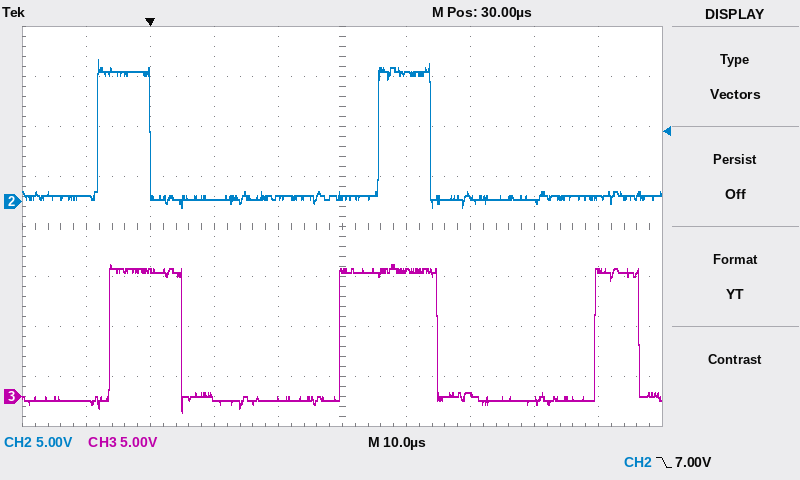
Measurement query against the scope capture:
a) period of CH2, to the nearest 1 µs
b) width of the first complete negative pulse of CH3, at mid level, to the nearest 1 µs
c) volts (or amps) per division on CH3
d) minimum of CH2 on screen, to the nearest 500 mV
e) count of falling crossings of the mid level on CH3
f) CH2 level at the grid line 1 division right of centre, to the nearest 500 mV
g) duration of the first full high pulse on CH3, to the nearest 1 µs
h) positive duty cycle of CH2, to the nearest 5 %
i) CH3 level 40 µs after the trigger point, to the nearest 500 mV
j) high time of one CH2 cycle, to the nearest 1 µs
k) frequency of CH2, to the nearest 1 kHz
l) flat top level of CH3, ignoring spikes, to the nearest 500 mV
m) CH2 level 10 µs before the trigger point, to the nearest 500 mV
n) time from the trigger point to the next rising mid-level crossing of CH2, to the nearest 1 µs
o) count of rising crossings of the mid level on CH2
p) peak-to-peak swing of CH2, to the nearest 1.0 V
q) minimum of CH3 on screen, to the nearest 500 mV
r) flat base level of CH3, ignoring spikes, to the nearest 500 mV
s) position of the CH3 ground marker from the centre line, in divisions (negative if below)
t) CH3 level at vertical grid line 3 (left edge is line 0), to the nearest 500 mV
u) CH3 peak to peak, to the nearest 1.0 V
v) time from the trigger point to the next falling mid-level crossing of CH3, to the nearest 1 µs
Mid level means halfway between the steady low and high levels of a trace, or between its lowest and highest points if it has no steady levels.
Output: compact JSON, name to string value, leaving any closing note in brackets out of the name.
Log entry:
{"period of CH2, to the nearest 1 µs": "44 µs", "width of the first complete negative pulse of CH3, at mid level, to the nearest 1 µs": "25 µs", "volts (or amps) per division on CH3": "5 V", "minimum of CH2 on screen, to the nearest 500 mV": "-500 mV", "count of falling crossings of the mid level on CH3": "3", "CH2 level at the grid line 1 division right of centre, to the nearest 500 mV": "13.0 V", "duration of the first full high pulse on CH3, to the nearest 1 µs": "11 µs", "positive duty cycle of CH2, to the nearest 5 %": "20 %", "CH3 level 40 µs after the trigger point, to the nearest 500 mV": "12.5 V", "high time of one CH2 cycle, to the nearest 1 µs": "8 µs", "frequency of CH2, to the nearest 1 kHz": "23 kHz", "flat top level of CH3, ignoring spikes, to the nearest 500 mV": "12.5 V", "CH2 level 10 µs before the trigger point, to the nearest 500 mV": "500 mV", "time from the trigger point to the next rising mid-level crossing of CH2, to the nearest 1 µs": "36 µs", "count of rising crossings of the mid level on CH2": "2", "peak-to-peak swing of CH2, to the nearest 1.0 V": "15.0 V", "minimum of CH3 on screen, to the nearest 500 mV": "-1.5 V", "flat base level of CH3, ignoring spikes, to the nearest 500 mV": "-500 mV", "position of the CH3 ground marker from the centre line, in divisions": "-3.4 div", "CH3 level at vertical grid line 3 (left edge is line 0), to the nearest 500 mV": "0.0 V", "CH3 peak to peak, to the nearest 1.0 V": "15.0 V", "time from the trigger point to the next falling mid-level crossing of CH3, to the nearest 1 µs": "5 µs"}
